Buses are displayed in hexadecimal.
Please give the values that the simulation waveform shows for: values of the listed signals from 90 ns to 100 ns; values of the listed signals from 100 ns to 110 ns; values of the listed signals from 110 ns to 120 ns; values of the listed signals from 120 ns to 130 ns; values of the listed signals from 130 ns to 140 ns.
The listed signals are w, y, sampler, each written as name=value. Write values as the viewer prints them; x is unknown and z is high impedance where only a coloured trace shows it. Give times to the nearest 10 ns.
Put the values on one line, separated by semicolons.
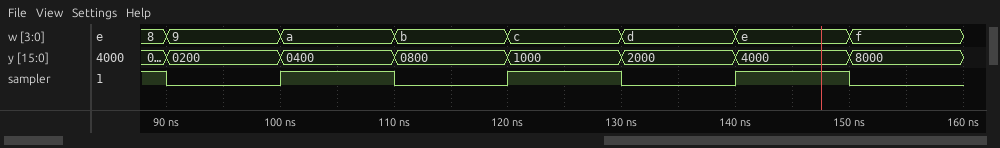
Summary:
w=9, y=0200, sampler=0; w=a, y=0400, sampler=1; w=b, y=0800, sampler=0; w=c, y=1000, sampler=1; w=d, y=2000, sampler=0
